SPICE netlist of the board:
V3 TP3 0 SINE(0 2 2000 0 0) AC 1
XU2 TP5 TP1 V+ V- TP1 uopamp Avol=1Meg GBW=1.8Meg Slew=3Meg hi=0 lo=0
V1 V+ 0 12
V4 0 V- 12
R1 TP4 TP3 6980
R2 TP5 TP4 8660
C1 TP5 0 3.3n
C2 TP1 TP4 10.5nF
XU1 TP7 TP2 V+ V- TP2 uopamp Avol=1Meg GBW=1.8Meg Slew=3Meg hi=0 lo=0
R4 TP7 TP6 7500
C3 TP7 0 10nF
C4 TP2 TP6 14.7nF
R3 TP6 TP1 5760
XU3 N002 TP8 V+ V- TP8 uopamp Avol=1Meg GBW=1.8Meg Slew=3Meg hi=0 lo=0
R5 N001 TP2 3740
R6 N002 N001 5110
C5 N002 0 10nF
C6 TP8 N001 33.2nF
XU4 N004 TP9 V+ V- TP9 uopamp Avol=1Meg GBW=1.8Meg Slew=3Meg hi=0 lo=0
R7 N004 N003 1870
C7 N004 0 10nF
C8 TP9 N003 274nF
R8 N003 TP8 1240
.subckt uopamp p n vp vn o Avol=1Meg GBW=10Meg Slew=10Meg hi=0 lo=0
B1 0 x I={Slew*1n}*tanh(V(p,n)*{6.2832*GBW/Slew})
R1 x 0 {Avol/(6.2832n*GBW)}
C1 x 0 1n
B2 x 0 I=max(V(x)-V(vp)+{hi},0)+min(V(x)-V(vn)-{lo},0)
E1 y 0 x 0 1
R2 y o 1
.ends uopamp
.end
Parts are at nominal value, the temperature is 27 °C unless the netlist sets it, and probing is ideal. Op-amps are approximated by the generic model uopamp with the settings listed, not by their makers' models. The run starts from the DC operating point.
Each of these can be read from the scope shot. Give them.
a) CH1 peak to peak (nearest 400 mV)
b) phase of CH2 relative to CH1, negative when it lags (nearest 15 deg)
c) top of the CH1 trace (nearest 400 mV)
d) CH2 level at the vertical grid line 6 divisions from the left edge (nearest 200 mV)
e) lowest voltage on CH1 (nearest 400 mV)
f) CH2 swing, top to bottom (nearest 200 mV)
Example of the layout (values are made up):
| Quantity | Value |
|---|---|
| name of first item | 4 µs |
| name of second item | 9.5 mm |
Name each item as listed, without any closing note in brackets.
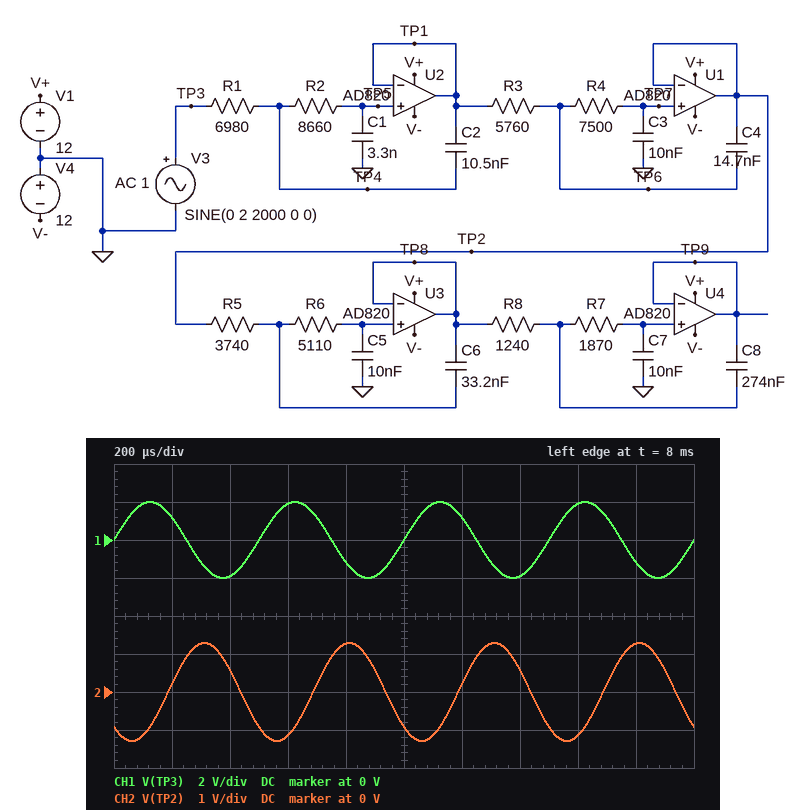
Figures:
| Quantity | Value |
|---|---|
| CH1 peak to peak | 4.0 V |
| phase of CH2 relative to CH1, negative when it lags | -135 deg |
| top of the CH1 trace | 2.0 V |
| CH2 level at the vertical grid line 6 divisions from the left edge | 200 mV |
| lowest voltage on CH1 | -2.0 V |
| CH2 swing, top to bottom | 2.6 V |
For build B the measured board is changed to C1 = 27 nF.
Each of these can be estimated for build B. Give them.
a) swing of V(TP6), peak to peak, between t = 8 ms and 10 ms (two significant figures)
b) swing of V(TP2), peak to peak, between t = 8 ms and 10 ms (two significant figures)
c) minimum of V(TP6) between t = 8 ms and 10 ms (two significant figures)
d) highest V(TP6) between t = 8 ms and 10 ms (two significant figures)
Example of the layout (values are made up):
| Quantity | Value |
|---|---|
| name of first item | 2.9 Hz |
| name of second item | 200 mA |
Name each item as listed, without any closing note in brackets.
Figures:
| Quantity | Value |
|---|---|
| swing of V(TP6), peak to peak, between t = 8 ms and 10 ms | 590 mV |
| swing of V(TP2), peak to peak, between t = 8 ms and 10 ms | 430 mV |
| minimum of V(TP6) between t = 8 ms and 10 ms | -300 mV |
| highest V(TP6) between t = 8 ms and 10 ms | 300 mV |
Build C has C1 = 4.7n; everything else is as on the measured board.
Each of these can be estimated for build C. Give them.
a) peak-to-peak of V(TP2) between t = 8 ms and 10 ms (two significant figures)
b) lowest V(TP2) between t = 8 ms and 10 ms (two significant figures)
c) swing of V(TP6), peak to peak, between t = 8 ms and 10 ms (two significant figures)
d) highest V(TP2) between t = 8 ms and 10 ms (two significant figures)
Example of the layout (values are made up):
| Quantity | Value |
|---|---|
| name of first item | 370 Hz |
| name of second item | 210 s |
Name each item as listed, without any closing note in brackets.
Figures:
| Quantity | Value |
|---|---|
| peak-to-peak of V(TP2) between t = 8 ms and 10 ms | 2.3 V |
| lowest V(TP2) between t = 8 ms and 10 ms | -1.1 V |
| swing of V(TP6), peak to peak, between t = 8 ms and 10 ms | 3.1 V |
| highest V(TP2) between t = 8 ms and 10 ms | 1.1 V |
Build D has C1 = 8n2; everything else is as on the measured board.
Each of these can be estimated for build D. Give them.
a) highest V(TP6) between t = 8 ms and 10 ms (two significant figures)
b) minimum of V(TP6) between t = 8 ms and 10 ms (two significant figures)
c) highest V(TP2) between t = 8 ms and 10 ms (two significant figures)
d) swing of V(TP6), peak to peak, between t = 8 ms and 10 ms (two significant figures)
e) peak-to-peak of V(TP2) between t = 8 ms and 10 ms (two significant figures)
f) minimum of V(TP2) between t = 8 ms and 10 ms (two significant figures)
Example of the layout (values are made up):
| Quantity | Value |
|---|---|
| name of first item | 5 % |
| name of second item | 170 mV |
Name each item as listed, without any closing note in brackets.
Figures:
| Quantity | Value |
|---|---|
| highest V(TP6) between t = 8 ms and 10 ms | 1.0 V |
| minimum of V(TP6) between t = 8 ms and 10 ms | -1.0 V |
| highest V(TP2) between t = 8 ms and 10 ms | 740 mV |
| swing of V(TP6), peak to peak, between t = 8 ms and 10 ms | 2.0 V |
| peak-to-peak of V(TP2) between t = 8 ms and 10 ms | 1.5 V |
| minimum of V(TP2) between t = 8 ms and 10 ms | -740 mV |
